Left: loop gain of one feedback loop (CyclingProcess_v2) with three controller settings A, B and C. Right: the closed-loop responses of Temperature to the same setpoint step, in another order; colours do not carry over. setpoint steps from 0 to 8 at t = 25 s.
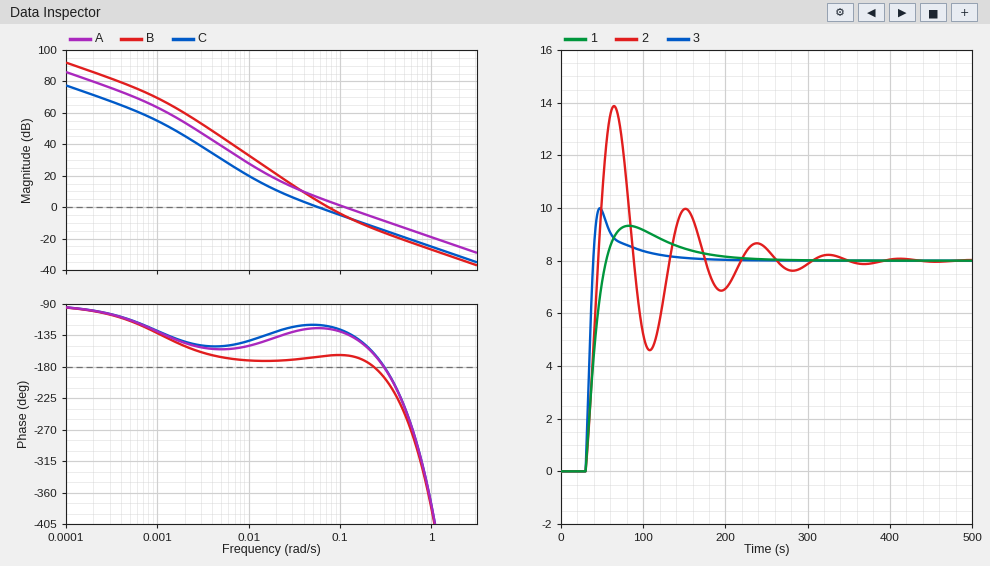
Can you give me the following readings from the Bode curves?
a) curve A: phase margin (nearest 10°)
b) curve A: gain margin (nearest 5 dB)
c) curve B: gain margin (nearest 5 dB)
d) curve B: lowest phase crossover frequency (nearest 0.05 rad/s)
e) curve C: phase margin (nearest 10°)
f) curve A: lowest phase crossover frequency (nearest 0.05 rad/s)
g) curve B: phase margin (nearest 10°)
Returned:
50°
10 dB
15 dB
0.25 rad/s
60°
0.30 rad/s
20°
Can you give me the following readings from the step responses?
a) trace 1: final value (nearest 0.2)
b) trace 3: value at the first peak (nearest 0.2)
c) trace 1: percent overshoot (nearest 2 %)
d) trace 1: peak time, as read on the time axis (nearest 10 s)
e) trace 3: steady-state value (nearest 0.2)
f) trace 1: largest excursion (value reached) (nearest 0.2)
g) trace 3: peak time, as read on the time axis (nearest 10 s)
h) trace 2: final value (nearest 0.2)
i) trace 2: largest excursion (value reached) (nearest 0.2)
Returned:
8.0
10.0
16 %
80 s
8.0
9.4
50 s
8.0
13.8
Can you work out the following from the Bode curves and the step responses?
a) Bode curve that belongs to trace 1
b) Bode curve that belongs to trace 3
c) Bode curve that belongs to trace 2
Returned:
C
A
B
